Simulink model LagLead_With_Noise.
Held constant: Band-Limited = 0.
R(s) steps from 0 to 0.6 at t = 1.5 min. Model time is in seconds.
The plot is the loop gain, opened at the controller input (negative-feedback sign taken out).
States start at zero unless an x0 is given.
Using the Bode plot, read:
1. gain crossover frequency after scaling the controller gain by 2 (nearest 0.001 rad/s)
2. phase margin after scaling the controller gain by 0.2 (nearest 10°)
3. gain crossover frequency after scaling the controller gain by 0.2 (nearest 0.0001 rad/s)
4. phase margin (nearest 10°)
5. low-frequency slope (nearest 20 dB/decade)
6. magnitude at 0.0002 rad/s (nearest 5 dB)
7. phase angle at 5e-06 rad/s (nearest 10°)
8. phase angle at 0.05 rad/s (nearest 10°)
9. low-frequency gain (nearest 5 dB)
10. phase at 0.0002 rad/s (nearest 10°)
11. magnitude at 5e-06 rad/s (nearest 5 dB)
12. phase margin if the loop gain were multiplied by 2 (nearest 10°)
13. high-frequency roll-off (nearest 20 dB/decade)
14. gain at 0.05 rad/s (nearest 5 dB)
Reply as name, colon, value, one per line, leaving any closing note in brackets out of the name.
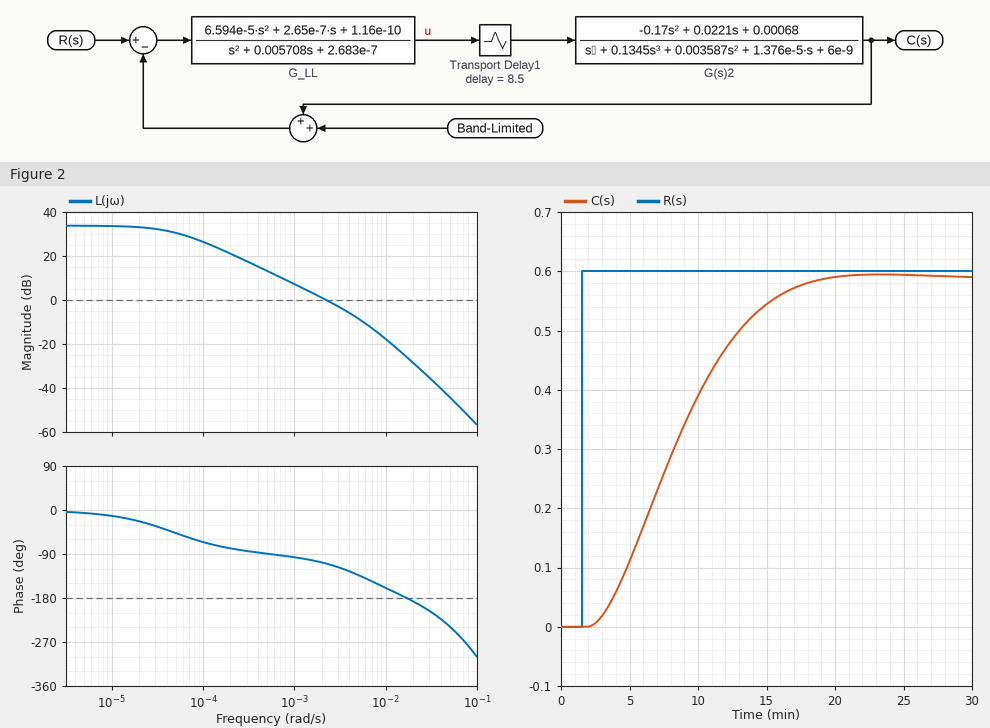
gain crossover frequency after scaling the controller gain by 2: 0.004 rad/s
phase margin after scaling the controller gain by 0.2: 90°
gain crossover frequency after scaling the controller gain by 0.2: 0.0005 rad/s
phase margin: 70°
low-frequency slope: 0 dB/decade
magnitude at 0.0002 rad/s: 20 dB
phase angle at 5e-06 rad/s: -10°
phase angle at 0.05 rad/s: -240°
low-frequency gain: 35 dB
phase at 0.0002 rad/s: -80°
magnitude at 5e-06 rad/s: 35 dB
phase margin if the loop gain were multiplied by 2: 50°
high-frequency roll-off: -40 dB/decade
gain at 0.05 rad/s: -45 dB
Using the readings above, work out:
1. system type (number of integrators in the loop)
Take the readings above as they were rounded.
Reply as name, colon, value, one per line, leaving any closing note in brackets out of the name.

system type: 0
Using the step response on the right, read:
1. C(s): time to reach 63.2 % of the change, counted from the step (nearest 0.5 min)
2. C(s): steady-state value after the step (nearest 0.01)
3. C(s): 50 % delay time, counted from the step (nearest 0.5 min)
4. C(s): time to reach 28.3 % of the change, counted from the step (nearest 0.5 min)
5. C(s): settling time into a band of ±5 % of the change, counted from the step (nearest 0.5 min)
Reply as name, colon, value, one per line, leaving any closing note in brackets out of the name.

C(s): time to reach 63.2 % of the change, counted from the step: 8.0 min
C(s): steady-state value after the step: 0.59
C(s): 50 % delay time, counted from the step: 6.5 min
C(s): time to reach 28.3 % of the change, counted from the step: 4.5 min
C(s): settling time into a band of ±5 % of the change, counted from the step: 14.5 min
